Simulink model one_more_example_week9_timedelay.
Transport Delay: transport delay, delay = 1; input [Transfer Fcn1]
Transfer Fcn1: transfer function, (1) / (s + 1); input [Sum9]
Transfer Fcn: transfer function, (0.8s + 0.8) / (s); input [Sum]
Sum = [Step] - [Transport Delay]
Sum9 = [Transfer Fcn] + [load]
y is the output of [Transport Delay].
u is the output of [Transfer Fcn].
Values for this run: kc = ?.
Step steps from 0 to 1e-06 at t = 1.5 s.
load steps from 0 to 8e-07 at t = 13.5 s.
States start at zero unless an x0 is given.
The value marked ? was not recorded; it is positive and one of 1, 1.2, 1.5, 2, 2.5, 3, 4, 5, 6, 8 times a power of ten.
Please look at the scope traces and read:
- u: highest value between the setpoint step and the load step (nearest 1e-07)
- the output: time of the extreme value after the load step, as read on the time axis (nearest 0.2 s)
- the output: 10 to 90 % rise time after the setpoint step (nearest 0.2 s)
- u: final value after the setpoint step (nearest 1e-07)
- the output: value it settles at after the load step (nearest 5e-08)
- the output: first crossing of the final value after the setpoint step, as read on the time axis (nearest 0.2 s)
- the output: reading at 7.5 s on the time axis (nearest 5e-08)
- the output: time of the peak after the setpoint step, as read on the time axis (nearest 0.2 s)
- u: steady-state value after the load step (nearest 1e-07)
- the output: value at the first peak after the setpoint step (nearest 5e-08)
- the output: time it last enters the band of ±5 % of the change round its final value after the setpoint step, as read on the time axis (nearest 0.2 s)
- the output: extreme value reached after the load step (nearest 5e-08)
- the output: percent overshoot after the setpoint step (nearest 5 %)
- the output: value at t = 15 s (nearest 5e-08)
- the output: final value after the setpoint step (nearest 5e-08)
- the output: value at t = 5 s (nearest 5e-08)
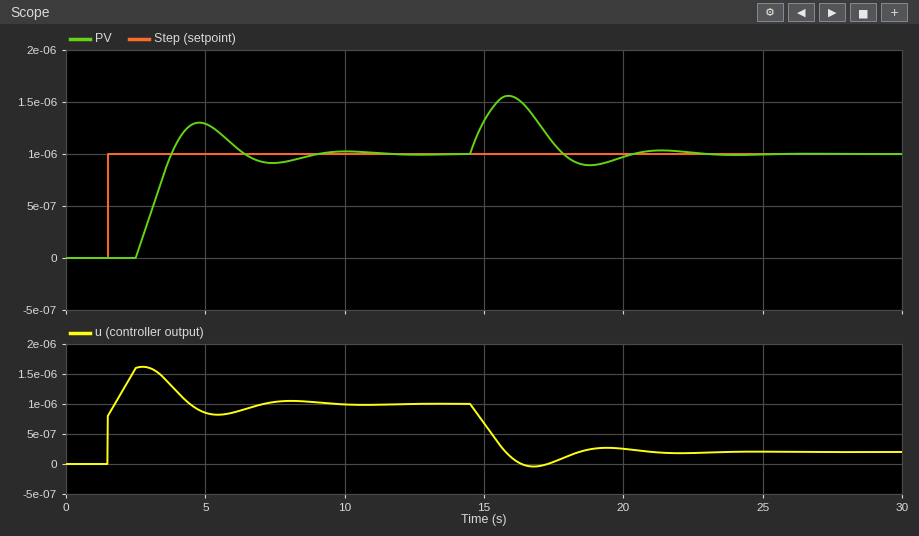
0.0000016
15.8 s
1.0 s
0.0000010
0.00000100
3.8 s
0.00000090
4.8 s
0.0000002
0.00000130
8.2 s
0.00000155
30 %
0.00000130
0.00000100
0.00000130
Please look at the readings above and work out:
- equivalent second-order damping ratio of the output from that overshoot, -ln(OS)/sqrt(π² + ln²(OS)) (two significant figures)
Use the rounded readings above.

0.36
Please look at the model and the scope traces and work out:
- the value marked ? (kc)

0.8
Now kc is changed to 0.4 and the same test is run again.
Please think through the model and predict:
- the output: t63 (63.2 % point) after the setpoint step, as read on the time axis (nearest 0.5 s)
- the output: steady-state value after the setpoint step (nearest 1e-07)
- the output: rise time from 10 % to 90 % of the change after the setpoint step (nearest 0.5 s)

4.0 s
0.0000010
3.0 s
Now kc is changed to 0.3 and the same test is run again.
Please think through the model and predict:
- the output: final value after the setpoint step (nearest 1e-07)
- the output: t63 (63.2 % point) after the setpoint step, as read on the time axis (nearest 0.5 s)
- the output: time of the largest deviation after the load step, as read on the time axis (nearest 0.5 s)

0.0000010
5.0 s
16.5 s
